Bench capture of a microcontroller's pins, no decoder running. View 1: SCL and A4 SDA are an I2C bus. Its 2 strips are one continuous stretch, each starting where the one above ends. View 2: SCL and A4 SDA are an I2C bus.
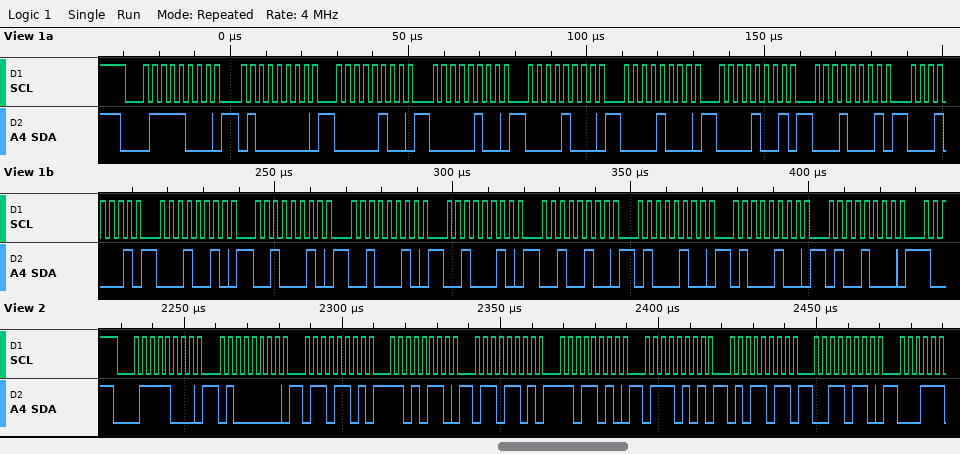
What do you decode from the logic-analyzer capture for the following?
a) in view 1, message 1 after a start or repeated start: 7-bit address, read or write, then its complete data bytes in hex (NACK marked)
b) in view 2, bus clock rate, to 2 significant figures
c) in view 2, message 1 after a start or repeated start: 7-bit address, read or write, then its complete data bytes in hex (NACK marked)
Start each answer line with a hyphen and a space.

- 0x3C write: 40 04 04 08 08 09 11 11 12 22 22 22 24 44 44 48
- 400 kHz
- 0x3C write: 40 6D D6 6D DA 75 5B 36
